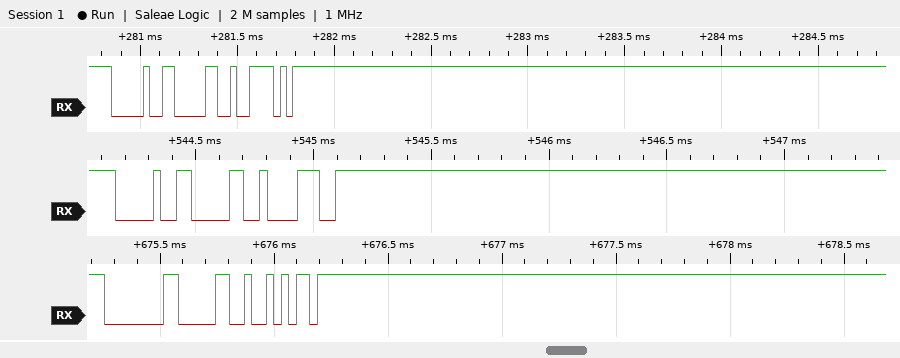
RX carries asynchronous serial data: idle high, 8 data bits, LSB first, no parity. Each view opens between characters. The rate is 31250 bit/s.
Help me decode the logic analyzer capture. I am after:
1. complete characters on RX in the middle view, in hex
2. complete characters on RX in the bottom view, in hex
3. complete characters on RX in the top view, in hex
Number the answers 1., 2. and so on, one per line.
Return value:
1. 90, 30, 38
2. 80, 30, 6A
3. 90, 30, 5E
